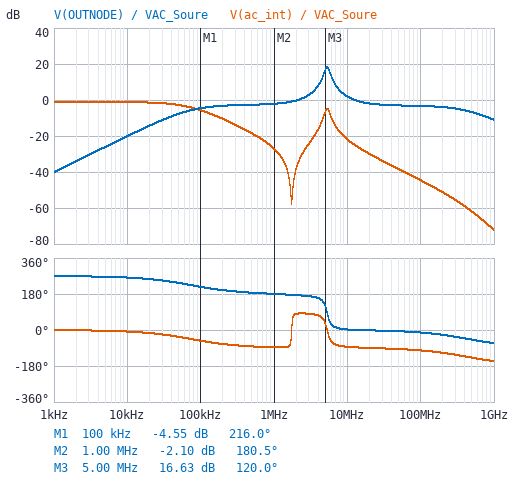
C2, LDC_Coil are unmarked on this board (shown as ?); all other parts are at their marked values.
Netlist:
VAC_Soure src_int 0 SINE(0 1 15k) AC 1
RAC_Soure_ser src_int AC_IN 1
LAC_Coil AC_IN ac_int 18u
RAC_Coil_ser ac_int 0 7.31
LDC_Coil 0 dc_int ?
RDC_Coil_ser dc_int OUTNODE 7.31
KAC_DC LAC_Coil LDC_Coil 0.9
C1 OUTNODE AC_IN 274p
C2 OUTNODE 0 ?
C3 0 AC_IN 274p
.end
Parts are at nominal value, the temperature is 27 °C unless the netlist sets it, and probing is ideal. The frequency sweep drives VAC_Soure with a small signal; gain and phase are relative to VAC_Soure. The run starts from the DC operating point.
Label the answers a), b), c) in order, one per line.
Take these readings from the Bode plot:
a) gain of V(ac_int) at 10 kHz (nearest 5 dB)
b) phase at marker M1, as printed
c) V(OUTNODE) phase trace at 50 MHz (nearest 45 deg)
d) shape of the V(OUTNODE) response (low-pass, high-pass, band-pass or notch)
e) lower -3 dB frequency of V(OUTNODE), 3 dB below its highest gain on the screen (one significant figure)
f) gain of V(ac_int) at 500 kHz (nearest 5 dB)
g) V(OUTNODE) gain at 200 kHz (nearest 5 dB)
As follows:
a) 0 dB
b) 216.0 deg
c) 0 deg
d) band-pass
e) 5 MHz
f) -20 dB
g) -5 dB
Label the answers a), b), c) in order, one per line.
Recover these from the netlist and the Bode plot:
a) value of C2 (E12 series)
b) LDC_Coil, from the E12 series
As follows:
a) 120 pF
b) 12 µH
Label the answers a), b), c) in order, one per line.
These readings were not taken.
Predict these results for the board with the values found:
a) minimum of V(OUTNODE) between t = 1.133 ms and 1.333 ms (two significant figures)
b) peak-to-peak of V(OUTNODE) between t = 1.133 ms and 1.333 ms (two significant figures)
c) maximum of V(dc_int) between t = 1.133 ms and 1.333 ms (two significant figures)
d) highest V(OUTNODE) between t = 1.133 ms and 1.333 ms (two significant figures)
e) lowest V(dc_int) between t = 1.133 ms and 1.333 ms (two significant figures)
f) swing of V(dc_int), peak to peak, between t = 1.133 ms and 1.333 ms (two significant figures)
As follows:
a) -150 mV
b) 290 mV
c) 150 mV
d) 150 mV
e) -150 mV
f) 290 mV
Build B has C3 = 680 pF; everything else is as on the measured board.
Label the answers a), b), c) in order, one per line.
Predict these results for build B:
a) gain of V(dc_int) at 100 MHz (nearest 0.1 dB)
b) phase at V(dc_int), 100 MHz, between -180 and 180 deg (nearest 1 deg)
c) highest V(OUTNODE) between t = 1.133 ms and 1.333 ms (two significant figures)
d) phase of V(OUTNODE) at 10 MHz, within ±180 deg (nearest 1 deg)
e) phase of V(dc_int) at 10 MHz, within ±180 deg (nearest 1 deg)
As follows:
a) -4.0 dB
b) -25 deg
c) 150 mV
d) 1 deg
e) 6 deg
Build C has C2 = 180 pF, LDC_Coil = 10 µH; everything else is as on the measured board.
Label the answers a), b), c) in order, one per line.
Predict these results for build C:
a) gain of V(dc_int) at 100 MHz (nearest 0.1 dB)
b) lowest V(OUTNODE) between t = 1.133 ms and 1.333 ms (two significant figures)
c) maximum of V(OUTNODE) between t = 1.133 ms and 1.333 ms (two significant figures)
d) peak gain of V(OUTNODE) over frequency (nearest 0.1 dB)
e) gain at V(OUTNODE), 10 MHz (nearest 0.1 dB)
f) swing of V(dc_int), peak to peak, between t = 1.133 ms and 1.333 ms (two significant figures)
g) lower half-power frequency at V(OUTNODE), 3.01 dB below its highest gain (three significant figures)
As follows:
a) -4.6 dB
b) -130 mV
c) 130 mV
d) 16.6 dB
e) 1.0 dB
f) 270 mV
g) 4.92 MHz
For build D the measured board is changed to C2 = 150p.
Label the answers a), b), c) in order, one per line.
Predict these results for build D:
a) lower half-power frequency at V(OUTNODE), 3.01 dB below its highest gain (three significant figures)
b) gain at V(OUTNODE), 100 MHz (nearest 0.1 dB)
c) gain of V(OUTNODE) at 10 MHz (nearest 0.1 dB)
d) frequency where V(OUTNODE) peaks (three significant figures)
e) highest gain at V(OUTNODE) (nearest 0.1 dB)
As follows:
a) 4.67 MHz
b) -4.0 dB
c) 1.1 dB
d) 5.11 MHz
e) 17.7 dB
